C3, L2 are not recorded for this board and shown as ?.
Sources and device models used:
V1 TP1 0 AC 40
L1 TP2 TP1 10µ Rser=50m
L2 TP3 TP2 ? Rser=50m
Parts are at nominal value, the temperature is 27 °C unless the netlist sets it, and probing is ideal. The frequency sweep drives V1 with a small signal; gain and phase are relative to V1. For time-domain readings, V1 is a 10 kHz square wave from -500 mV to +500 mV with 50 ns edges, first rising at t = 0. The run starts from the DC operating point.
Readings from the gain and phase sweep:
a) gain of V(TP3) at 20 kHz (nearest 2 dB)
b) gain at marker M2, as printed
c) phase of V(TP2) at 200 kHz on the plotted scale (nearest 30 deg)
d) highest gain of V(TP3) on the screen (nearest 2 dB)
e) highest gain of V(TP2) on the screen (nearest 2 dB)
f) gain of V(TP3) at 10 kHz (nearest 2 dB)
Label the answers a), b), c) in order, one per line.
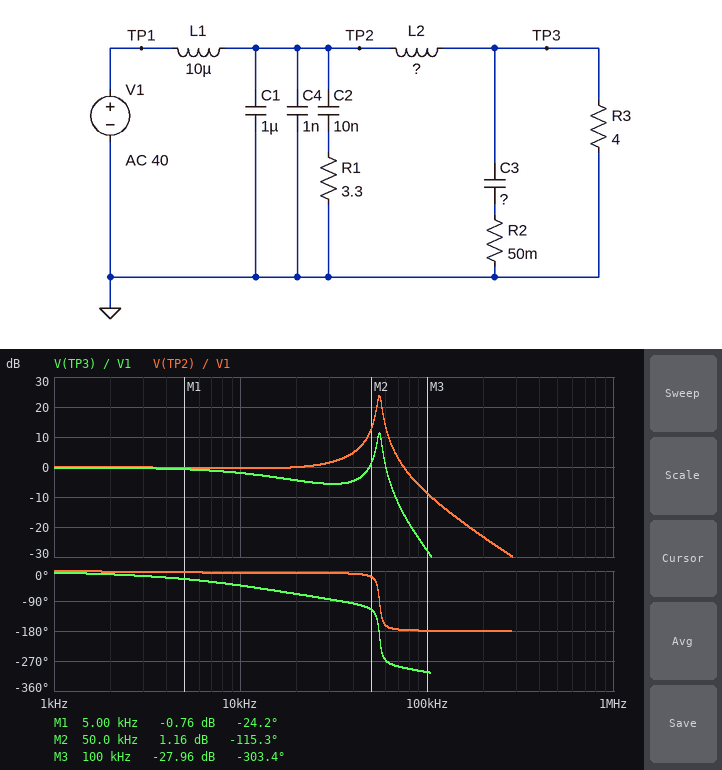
a) -4 dB
b) 1.16 dB
c) -180 deg
d) 12 dB
e) 24 dB
f) -2 dB
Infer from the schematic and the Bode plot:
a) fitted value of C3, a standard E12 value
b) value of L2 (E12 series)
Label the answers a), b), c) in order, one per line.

a) 330 nF
b) 47 µH
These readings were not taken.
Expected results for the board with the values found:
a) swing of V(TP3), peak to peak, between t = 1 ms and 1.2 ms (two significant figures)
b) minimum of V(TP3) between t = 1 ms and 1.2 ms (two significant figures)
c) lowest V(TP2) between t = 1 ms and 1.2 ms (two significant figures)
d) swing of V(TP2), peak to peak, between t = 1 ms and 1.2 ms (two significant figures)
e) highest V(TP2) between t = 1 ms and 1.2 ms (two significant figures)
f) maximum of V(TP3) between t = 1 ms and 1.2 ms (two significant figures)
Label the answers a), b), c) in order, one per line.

a) 1.1 V
b) -570 mV
c) -1.0 V
d) 2.0 V
e) 1.0 V
f) 570 mV
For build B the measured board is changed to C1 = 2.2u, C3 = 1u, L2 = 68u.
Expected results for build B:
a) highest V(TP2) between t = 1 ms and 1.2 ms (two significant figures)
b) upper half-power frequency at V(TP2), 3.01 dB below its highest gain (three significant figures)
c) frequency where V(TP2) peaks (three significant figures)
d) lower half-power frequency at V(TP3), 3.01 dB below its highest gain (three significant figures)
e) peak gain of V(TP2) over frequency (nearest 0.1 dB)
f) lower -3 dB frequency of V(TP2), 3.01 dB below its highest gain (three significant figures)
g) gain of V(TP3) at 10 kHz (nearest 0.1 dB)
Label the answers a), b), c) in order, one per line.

a) 960 mV
b) 37.3 kHz
c) 36.5 kHz
d) 35.7 kHz
e) 26.3 dB
f) 35.8 kHz
g) -2.4 dB
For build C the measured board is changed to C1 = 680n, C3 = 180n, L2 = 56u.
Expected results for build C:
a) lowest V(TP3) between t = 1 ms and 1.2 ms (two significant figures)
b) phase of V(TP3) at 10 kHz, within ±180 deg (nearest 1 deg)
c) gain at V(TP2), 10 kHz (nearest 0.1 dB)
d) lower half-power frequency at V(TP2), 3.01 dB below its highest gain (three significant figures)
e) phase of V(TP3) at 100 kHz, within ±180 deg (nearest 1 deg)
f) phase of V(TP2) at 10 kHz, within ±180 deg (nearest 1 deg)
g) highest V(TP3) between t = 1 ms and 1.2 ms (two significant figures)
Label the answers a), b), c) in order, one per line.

a) -530 mV
b) -47 deg
c) -0.5 dB
d) 64.6 kHz
e) 73 deg
f) -5 deg
g) 530 mV
